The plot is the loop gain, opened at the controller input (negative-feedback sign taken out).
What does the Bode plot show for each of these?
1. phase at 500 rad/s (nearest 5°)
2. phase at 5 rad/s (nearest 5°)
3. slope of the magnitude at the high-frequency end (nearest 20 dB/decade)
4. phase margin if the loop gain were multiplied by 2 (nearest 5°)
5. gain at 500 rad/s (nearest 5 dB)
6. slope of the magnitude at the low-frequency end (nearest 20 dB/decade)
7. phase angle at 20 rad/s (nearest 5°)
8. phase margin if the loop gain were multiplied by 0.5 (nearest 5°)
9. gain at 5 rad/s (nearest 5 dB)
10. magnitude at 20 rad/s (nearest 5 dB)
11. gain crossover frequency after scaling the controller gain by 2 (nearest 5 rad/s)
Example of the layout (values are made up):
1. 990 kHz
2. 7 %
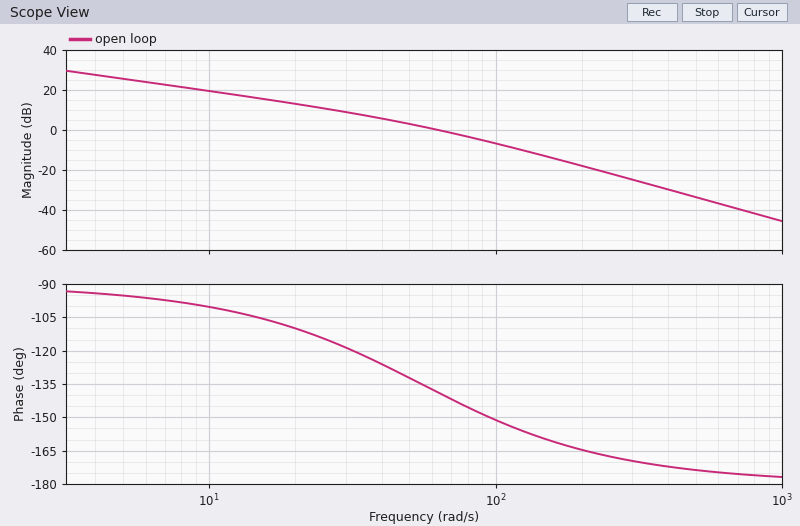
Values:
1. -175°
2. -95°
3. -40 dB/decade
4. 30°
5. -35 dB
6. -20 dB/decade
7. -110°
8. 55°
9. 25 dB
10. 15 dB
11. 95 rad/s
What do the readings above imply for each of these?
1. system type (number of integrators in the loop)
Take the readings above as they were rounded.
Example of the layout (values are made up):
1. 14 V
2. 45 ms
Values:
1. 1
